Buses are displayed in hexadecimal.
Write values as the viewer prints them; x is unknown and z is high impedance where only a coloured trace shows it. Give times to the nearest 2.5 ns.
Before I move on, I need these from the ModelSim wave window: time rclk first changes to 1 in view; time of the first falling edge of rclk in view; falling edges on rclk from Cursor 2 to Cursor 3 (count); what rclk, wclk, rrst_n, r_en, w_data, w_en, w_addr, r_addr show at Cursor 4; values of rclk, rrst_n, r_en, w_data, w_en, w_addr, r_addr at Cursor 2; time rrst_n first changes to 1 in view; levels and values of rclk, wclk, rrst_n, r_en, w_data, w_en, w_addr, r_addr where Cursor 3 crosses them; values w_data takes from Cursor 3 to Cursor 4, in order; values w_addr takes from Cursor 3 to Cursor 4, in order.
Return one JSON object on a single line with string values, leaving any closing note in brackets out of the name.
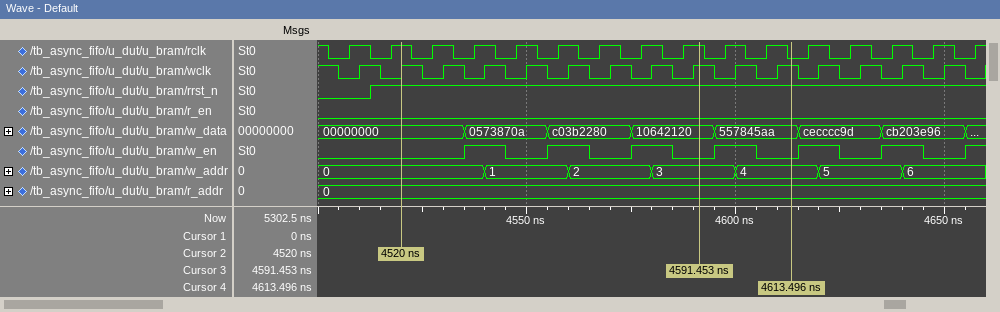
{"time rclk first changes to 1 in view": "4507.5 ns", "time of the first falling edge of rclk in view": "4502.5 ns", "falling edges on rclk from Cursor 2 to Cursor 3": "7", "what rclk, wclk, rrst_n, r_en, w_data, w_en, w_addr, r_addr show at Cursor 4": "rclk=0, wclk=1, rrst_n=1, r_en=0, w_data=557845aa, w_en=0, w_addr=4, r_addr=0", "values of rclk, rrst_n, r_en, w_data, w_en, w_addr, r_addr at Cursor 2": "rclk=1, rrst_n=1, r_en=0, w_data=00000000, w_en=0, w_addr=0, r_addr=0", "time rrst_n first changes to 1 in view": "4512.5 ns", "levels and values of rclk, wclk, rrst_n, r_en, w_data, w_en, w_addr, r_addr where Cursor 3 crosses them": "rclk=1, wclk=1, rrst_n=1, r_en=0, w_data=10642120, w_en=0, w_addr=3, r_addr=0", "values w_data takes from Cursor 3 to Cursor 4, in order": "10642120, 557845aa", "values w_addr takes from Cursor 3 to Cursor 4, in order": "3, 4"}
